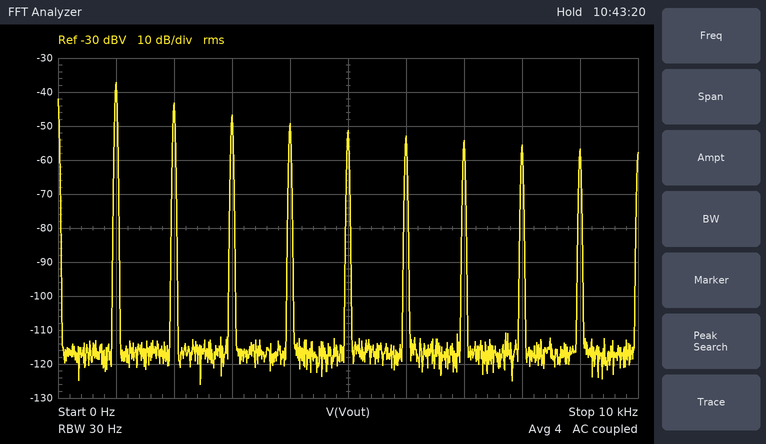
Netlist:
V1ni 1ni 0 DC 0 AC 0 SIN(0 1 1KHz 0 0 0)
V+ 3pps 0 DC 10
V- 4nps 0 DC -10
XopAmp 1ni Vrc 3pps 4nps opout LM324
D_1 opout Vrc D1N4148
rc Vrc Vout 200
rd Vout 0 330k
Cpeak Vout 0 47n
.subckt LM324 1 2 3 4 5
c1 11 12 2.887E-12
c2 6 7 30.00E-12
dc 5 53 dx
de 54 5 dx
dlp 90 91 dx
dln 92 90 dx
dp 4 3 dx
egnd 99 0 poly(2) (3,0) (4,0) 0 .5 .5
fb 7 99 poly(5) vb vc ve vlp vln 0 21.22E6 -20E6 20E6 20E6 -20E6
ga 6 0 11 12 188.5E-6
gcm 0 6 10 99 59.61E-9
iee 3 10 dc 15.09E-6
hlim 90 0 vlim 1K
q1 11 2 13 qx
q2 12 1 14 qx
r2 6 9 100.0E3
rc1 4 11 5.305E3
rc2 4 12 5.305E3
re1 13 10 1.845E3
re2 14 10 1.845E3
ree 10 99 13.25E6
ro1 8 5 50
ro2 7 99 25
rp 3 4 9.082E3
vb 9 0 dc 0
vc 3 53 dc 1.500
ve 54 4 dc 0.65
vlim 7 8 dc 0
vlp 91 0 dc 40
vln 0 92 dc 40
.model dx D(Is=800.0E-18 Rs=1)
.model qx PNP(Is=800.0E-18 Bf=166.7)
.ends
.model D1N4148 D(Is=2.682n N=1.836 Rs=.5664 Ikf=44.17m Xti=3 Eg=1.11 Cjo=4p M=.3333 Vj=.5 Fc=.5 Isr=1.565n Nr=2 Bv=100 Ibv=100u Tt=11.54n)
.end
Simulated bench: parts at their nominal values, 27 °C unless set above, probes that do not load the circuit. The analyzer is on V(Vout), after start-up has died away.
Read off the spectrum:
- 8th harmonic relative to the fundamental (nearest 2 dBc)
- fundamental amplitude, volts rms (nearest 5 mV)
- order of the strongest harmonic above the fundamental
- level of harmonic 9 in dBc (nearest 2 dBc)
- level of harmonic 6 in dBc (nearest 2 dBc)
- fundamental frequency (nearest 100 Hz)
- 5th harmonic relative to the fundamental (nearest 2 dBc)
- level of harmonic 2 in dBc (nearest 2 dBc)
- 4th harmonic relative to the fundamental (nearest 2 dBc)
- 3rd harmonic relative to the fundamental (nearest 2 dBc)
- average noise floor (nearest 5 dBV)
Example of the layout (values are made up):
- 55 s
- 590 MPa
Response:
- -18 dBc
- 15 mV
- 2
- -20 dBc
- -16 dBc
- 1.0 kHz
- -14 dBc
- -6 dBc
- -12 dBc
- -10 dBc
- -115 dBV
